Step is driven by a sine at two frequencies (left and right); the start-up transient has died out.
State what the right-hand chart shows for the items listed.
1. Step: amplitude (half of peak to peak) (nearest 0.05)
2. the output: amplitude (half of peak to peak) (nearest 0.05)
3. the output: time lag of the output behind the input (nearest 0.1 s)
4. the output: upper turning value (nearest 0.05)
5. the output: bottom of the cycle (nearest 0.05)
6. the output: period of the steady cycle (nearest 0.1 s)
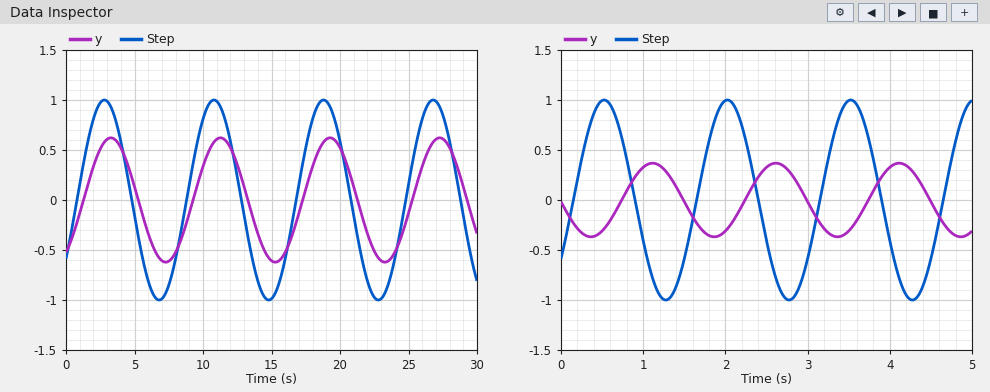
1.00
0.35
0.6 s
0.35
-0.35
1.5 s
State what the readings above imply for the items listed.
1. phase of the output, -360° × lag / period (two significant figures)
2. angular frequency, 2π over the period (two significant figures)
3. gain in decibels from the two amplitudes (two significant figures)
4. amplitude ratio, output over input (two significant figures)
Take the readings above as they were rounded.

-140°
4.2 rad/s
-9.1 dB
0.35
